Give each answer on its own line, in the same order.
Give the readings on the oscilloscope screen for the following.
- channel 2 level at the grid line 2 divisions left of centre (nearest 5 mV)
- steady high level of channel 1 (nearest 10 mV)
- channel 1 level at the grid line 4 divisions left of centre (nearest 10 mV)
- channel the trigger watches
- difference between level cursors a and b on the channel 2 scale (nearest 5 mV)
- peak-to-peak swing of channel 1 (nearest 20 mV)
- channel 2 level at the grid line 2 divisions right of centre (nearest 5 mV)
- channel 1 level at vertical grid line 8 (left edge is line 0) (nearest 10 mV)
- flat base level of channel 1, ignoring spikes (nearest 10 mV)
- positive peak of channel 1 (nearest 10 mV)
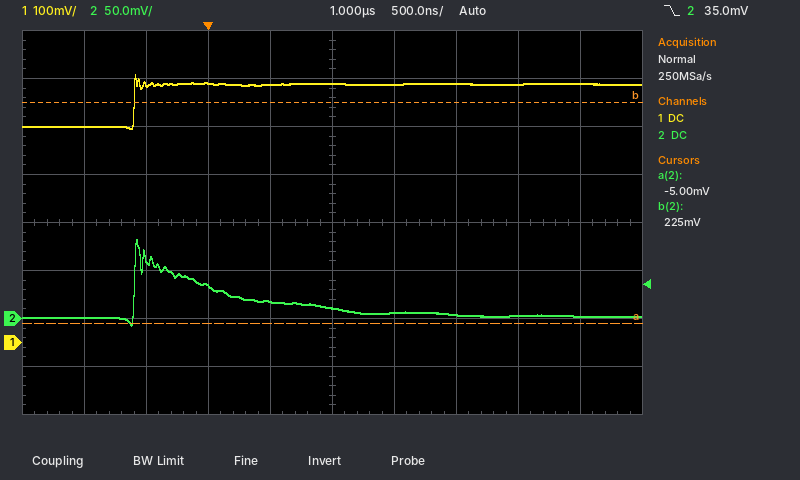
35 mV
540 mV
450 mV
channel 2
230 mV
120 mV
5 mV
540 mV
450 mV
560 mV
